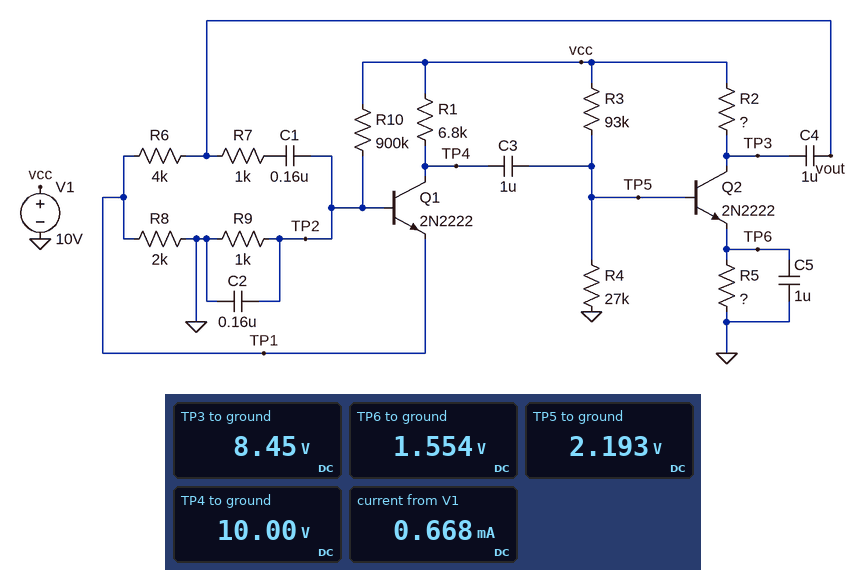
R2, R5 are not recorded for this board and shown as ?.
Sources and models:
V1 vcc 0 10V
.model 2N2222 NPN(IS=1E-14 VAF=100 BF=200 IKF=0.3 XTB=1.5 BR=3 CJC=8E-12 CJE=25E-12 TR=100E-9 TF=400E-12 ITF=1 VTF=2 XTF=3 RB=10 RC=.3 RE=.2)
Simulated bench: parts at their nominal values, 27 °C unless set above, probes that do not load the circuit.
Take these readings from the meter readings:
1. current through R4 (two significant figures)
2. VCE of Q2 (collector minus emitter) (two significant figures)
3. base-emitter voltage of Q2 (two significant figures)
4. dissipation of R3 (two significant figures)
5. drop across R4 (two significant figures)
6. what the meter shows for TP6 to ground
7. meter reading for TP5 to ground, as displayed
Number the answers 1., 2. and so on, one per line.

1. 81 µA
2. 6.9 V
3. 640 mV
4. 660 µW
5. 2.2 V
6. 1.554 V
7. 2.193 V
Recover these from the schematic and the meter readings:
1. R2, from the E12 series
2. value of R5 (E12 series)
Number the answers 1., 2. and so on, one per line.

1. 2.7 kΩ
2. 2.7 kΩ
